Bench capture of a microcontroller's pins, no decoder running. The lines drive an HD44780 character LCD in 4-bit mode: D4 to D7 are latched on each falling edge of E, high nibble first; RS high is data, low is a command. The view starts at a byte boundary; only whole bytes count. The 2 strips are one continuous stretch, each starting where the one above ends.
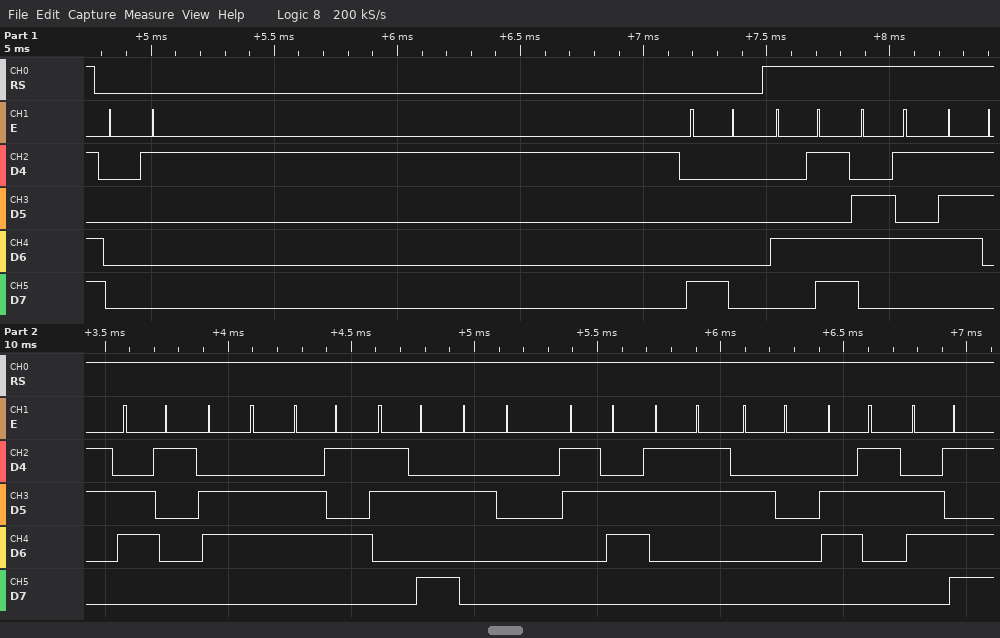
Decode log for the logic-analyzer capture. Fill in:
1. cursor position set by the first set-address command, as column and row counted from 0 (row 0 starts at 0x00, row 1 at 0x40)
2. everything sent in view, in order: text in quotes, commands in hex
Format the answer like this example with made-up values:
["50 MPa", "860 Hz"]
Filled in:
["column 0, row 0", "0x01 0x80 \"Mesafe: 63 cm\""]
